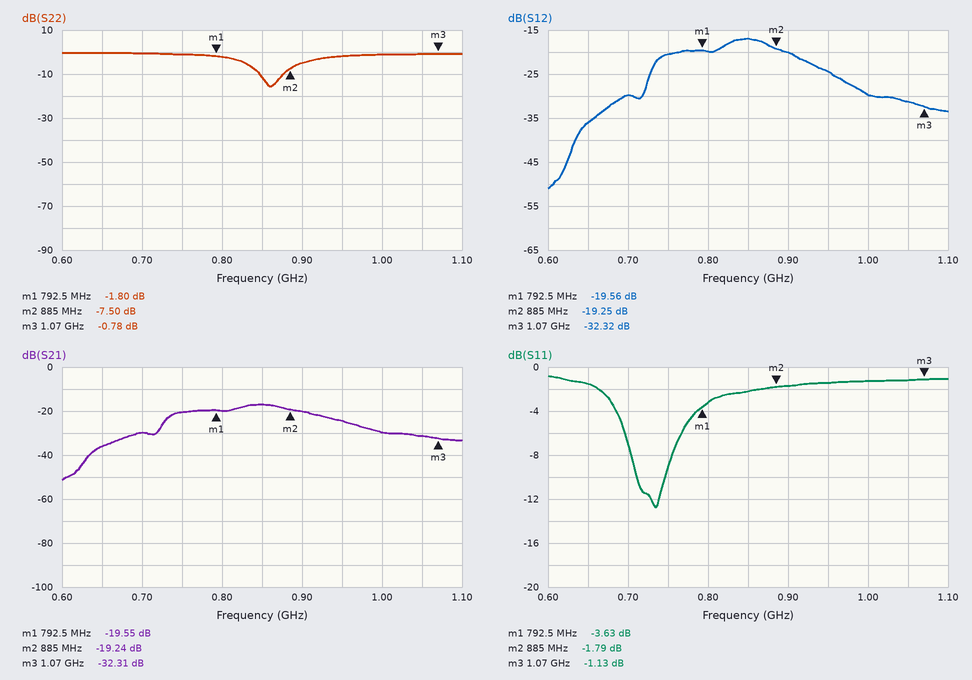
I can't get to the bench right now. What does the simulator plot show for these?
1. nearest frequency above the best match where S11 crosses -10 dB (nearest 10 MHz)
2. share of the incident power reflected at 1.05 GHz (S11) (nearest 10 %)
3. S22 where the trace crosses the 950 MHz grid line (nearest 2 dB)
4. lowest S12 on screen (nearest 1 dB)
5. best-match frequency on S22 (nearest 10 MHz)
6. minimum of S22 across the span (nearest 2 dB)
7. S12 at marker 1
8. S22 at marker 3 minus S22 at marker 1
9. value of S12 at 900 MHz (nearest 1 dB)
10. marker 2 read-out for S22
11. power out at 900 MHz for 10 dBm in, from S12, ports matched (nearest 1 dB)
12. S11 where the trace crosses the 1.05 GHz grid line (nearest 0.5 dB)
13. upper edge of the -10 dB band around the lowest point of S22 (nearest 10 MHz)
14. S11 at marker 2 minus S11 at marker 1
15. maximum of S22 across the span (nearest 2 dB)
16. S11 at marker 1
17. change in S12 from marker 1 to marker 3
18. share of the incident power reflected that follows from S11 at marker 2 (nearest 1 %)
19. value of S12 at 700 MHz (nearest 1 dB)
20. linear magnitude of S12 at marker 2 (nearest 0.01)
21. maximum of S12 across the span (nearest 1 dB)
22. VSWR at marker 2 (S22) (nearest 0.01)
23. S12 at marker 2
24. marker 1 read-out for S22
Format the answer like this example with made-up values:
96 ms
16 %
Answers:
750 MHz
80 %
-2 dB
-51 dB
860 MHz
-16 dB
-19.56 dB
1.02 dB
-20 dB
-7.50 dB
-10 dBm
-1.0 dB
880 MHz
1.84 dB
0 dB
-3.63 dB
-12.76 dB
66 %
-30 dB
0.11
-17 dB
2.46
-19.25 dB
-1.80 dB
